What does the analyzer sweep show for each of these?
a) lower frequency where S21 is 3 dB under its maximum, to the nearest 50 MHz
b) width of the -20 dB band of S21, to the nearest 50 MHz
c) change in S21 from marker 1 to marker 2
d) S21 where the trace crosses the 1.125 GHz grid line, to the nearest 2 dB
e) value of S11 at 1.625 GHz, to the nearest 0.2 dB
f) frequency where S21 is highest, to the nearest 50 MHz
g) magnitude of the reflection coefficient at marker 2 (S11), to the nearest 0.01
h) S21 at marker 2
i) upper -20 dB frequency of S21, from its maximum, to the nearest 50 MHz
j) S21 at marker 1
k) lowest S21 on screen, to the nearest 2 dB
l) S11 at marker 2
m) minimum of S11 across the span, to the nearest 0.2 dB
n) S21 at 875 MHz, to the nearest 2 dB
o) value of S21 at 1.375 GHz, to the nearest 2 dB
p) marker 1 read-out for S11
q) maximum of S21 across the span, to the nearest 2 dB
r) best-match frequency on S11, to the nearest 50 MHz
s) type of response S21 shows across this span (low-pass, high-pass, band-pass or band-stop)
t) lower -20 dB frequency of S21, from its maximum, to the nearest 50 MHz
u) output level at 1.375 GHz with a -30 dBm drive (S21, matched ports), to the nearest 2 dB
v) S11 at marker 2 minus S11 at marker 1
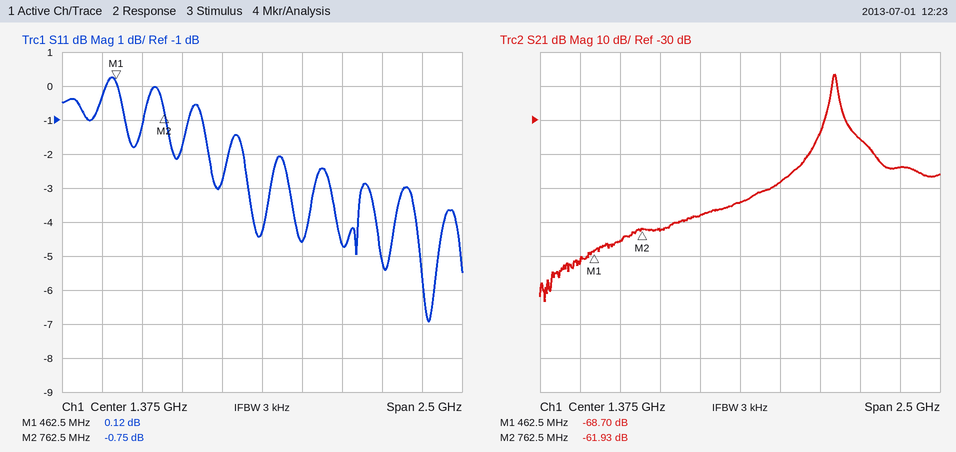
1.95 GHz
300 MHz
6.77 dB
-58 dB
-4.6 dB
1.95 GHz
0.92
-61.93 dB
2.15 GHz
-68.70 dB
-84 dB
-0.75 dB
-7.0 dB
-62 dB
-54 dB
0.12 dB
-16 dB
2.40 GHz
band-pass
1.85 GHz
-84 dBm
-0.87 dB
